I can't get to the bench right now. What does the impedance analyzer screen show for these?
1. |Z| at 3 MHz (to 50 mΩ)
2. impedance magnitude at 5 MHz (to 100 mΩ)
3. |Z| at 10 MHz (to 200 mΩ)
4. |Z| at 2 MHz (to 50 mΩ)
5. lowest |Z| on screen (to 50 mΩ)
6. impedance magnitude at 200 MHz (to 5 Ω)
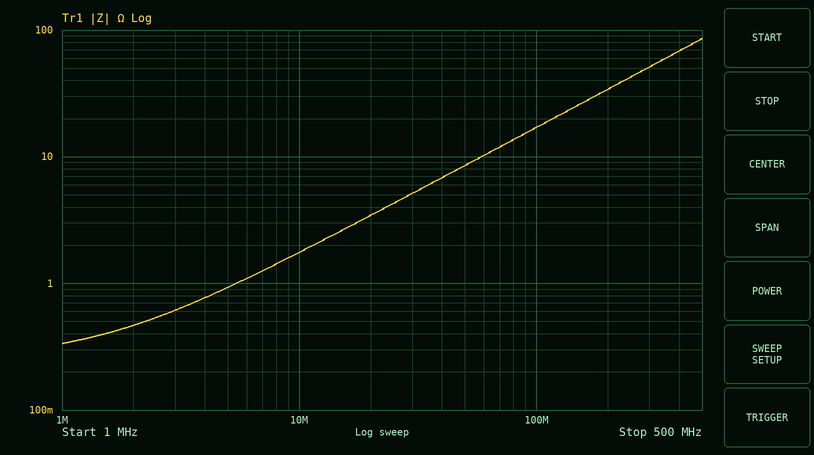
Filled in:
600 mΩ
900 mΩ
1.8 Ω
450 mΩ
350 mΩ
35 Ω
